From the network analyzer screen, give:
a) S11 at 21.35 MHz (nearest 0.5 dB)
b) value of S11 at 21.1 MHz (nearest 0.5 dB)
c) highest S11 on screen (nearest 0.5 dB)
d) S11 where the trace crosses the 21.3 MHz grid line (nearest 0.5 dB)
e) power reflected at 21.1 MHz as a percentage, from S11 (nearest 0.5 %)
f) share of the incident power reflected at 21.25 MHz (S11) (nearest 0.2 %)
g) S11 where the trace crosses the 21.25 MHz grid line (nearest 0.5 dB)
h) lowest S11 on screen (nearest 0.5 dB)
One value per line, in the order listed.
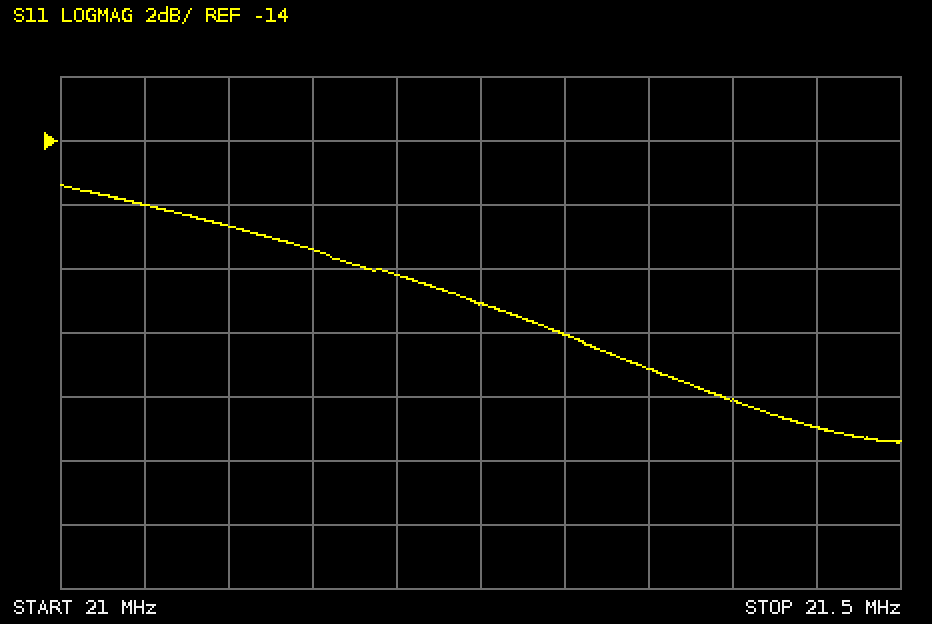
-21.0 dB
-16.5 dB
-15.5 dB
-20.0 dB
2.0 %
1.2 %
-19.0 dB
-23.5 dB
